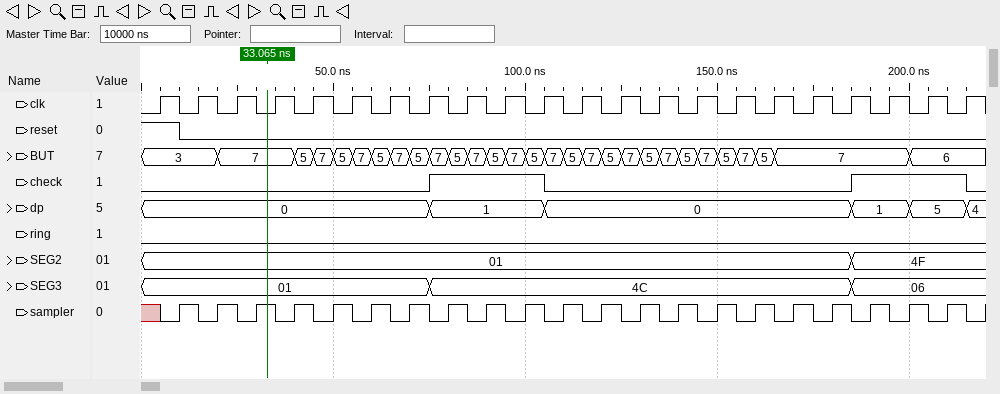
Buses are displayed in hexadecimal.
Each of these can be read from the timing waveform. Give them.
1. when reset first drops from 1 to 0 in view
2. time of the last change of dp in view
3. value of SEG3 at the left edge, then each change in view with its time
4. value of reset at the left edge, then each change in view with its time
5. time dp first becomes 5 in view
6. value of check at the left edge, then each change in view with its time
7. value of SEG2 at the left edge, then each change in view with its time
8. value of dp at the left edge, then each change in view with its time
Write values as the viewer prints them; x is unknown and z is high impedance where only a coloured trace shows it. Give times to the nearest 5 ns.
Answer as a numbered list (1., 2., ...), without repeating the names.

1. 10 ns
2. 215 ns
3. 01, 4C at 75 ns, 06 at 185 ns
4. 1, 0 at 10 ns
5. 200 ns
6. 0, 1 at 75 ns, 0 at 105 ns, 1 at 185 ns, 0 at 215 ns
7. 01, 4F at 185 ns
8. 0, 1 at 75 ns, 0 at 105 ns, 1 at 185 ns, 5 at 200 ns, 4 at 215 ns
